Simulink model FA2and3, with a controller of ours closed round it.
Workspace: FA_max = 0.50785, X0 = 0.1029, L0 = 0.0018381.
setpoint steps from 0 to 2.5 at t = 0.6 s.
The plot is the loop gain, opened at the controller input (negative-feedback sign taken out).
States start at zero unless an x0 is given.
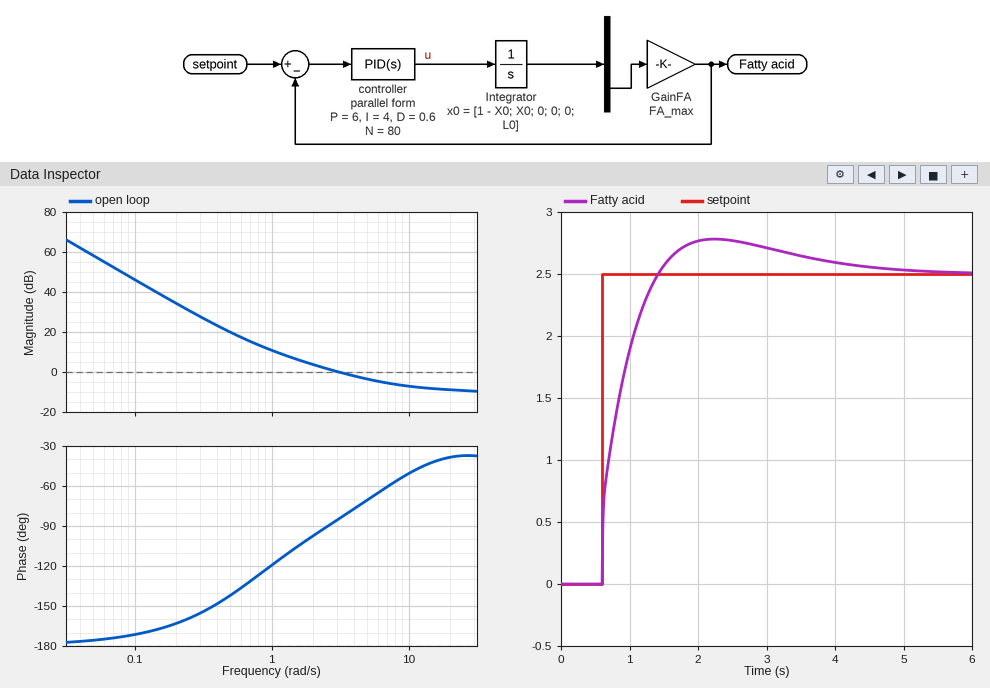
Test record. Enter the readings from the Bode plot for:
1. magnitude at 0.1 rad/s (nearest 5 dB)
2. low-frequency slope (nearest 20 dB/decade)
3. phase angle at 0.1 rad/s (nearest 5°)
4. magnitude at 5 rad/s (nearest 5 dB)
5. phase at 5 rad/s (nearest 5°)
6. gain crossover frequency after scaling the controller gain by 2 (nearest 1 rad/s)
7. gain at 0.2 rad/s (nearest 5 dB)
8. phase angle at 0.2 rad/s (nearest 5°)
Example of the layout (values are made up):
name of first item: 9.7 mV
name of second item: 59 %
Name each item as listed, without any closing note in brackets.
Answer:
magnitude at 0.1 rad/s: 45 dB
low-frequency slope: -40 dB/decade
phase angle at 0.1 rad/s: -170°
magnitude at 5 rad/s: -5 dB
phase at 5 rad/s: -70°
gain crossover frequency after scaling the controller gain by 2: 8 rad/s
gain at 0.2 rad/s: 35 dB
phase angle at 0.2 rad/s: -165°
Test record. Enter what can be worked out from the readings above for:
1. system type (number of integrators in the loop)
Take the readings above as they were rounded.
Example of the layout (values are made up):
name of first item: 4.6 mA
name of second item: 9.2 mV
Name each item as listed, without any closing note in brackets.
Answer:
system type: 2
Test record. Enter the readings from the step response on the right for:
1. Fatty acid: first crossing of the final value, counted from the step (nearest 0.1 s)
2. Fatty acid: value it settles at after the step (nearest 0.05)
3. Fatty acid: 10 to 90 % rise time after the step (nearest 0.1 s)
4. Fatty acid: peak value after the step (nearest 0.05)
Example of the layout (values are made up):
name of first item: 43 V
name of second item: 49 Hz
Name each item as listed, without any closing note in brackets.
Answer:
Fatty acid: first crossing of the final value, counted from the step: 0.8 s
Fatty acid: value it settles at after the step: 2.50
Fatty acid: 10 to 90 % rise time after the step: 0.6 s
Fatty acid: peak value after the step: 2.80
